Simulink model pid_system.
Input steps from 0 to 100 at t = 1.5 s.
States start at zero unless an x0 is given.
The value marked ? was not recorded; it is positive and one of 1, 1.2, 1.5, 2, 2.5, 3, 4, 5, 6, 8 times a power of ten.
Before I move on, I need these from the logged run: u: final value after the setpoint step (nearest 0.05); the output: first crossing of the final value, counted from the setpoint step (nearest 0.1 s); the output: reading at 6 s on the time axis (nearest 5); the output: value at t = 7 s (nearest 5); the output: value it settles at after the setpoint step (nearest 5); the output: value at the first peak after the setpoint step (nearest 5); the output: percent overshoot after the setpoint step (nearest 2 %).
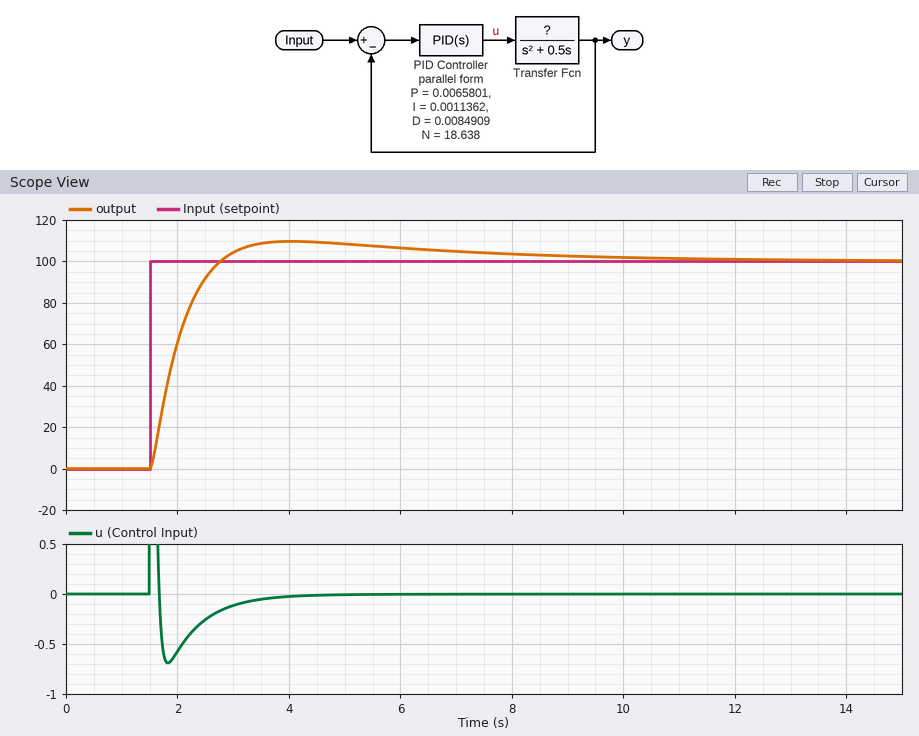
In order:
0.00
1.3 s
105
105
100
110
10 %
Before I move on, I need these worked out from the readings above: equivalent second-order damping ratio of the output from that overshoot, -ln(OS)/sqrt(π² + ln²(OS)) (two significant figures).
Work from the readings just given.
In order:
0.59
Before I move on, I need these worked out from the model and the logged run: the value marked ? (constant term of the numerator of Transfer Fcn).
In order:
200
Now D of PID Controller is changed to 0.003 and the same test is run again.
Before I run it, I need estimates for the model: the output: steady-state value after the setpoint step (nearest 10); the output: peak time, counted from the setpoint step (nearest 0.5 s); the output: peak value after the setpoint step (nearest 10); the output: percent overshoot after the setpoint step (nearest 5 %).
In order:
100
2.5 s
130
35 %
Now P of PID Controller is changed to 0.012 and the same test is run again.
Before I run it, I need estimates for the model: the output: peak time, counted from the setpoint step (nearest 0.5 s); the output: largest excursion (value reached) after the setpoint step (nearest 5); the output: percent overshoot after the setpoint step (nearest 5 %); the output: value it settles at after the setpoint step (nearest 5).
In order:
1.5 s
115
15 %
100
